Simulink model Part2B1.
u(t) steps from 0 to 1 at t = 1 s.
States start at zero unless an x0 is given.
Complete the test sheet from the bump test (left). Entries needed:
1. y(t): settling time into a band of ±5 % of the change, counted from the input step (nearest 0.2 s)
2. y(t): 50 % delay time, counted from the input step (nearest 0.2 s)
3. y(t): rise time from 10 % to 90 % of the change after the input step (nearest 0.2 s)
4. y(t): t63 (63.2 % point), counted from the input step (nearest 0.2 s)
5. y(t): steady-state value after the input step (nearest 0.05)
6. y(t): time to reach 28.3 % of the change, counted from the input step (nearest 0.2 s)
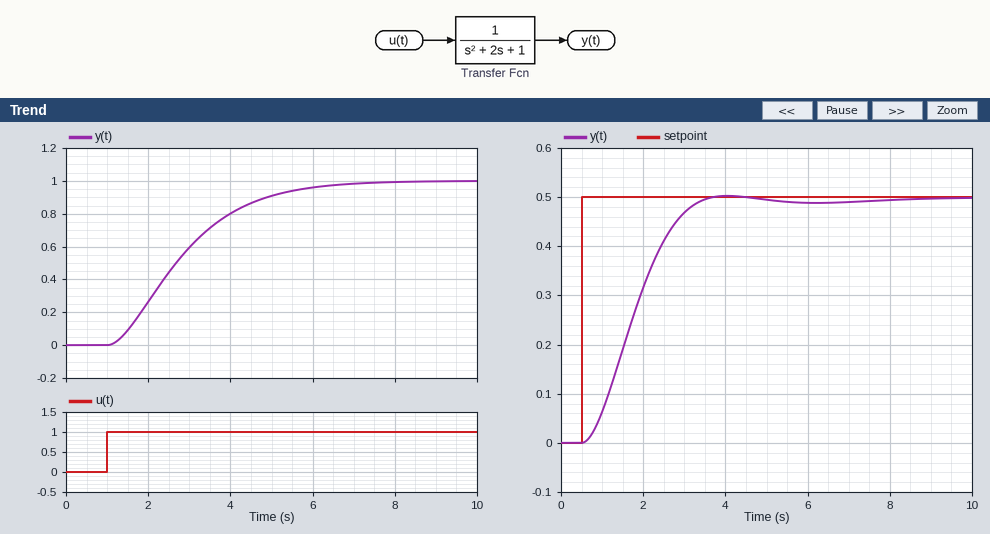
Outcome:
4.8 s
1.6 s
3.4 s
2.2 s
1.00
1.0 s
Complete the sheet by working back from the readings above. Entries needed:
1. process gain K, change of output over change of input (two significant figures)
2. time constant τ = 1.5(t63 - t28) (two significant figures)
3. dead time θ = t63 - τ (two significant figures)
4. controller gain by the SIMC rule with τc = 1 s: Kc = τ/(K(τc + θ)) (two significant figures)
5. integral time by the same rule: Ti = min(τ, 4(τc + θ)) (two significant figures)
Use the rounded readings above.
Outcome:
1.0
1.8 s
0.40 s
1.3
1.8 s
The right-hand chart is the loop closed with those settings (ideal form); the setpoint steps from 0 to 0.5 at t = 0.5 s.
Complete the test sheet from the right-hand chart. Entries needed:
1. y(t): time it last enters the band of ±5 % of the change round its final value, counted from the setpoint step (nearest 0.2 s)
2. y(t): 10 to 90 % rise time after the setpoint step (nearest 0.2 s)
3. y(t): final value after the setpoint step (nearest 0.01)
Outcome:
2.6 s
1.8 s
0.50
